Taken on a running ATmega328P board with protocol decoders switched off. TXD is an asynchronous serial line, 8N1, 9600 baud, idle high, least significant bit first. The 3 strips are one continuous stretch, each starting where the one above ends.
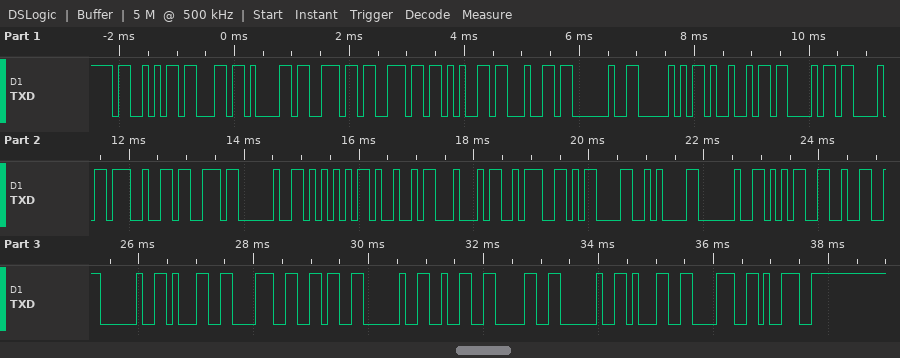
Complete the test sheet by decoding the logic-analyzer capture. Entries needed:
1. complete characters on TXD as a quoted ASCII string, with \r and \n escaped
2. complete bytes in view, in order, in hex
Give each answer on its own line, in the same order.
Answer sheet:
"Scanned PICC's UID:\r\n 52 186 20 189"
53 63 61 6E 6E 65 64 20 50 49 43 43 27 73 20 55 49 44 3A 0D 0A 20 35 32 20 31 38 36 20 32 30 20 31 38 39
